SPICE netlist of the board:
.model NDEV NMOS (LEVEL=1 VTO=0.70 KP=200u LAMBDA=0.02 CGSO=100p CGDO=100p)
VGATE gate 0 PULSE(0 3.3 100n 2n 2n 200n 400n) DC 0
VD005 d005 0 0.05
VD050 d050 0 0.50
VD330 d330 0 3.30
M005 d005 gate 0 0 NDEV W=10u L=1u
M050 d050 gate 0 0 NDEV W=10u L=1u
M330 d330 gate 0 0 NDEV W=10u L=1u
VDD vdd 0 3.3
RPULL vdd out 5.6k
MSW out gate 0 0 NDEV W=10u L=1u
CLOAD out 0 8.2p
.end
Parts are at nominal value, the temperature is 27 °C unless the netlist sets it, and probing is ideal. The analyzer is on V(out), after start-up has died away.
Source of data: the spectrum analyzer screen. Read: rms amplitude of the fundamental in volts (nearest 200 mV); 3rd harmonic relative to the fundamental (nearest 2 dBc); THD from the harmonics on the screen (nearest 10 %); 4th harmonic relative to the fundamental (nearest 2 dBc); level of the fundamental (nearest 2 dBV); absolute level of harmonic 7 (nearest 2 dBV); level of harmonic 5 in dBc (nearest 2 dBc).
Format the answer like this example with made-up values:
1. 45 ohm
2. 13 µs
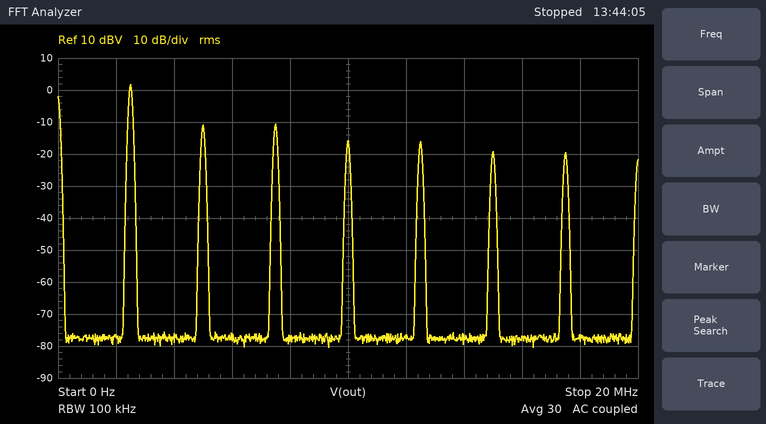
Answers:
1. 1.2 V
2. -12 dBc
3. 40 %
4. -18 dBc
5. 2 dBV
6. -20 dBV
7. -18 dBc
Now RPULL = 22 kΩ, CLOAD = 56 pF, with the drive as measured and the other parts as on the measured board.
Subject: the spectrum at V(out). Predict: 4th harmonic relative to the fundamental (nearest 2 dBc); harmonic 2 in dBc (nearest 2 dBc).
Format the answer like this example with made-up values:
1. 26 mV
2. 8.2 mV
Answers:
1. -16 dBc
2. -8 dBc
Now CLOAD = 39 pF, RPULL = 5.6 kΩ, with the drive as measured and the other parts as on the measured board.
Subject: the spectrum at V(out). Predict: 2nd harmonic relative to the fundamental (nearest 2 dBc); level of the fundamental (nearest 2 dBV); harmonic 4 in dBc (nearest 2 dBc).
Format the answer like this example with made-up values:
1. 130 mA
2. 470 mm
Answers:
1. -10 dBc
2. -4 dBV
3. -16 dBc
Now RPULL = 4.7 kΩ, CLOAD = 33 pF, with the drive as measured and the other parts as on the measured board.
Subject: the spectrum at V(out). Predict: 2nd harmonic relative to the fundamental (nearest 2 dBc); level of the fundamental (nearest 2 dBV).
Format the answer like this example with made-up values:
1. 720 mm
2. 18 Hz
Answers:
1. -10 dBc
2. -2 dBV
